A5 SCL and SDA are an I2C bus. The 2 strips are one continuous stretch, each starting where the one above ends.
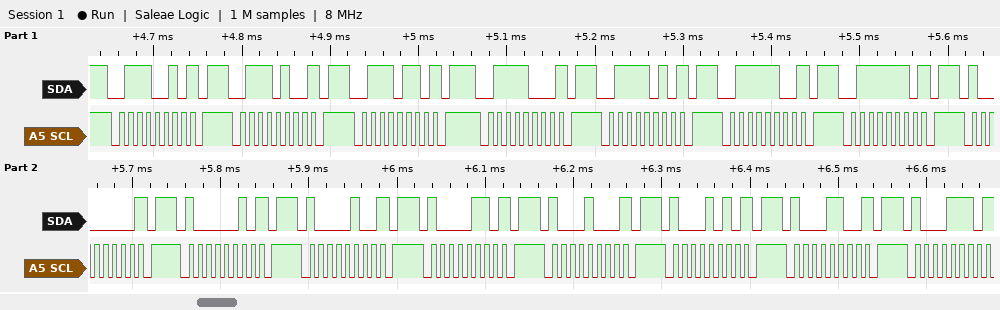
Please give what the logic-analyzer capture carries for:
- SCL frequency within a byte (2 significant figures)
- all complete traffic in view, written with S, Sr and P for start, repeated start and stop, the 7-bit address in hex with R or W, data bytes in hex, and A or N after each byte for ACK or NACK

100 kHz
S 39W N P S 3AW N P S 3BW N P S 3CW N P S 3DW N P S 3EW N P S 3FW N P S 40W N P S 41W N P S 42W N P S 43W N P S 44W N P S 45W N P S 46W N P S 47W N
